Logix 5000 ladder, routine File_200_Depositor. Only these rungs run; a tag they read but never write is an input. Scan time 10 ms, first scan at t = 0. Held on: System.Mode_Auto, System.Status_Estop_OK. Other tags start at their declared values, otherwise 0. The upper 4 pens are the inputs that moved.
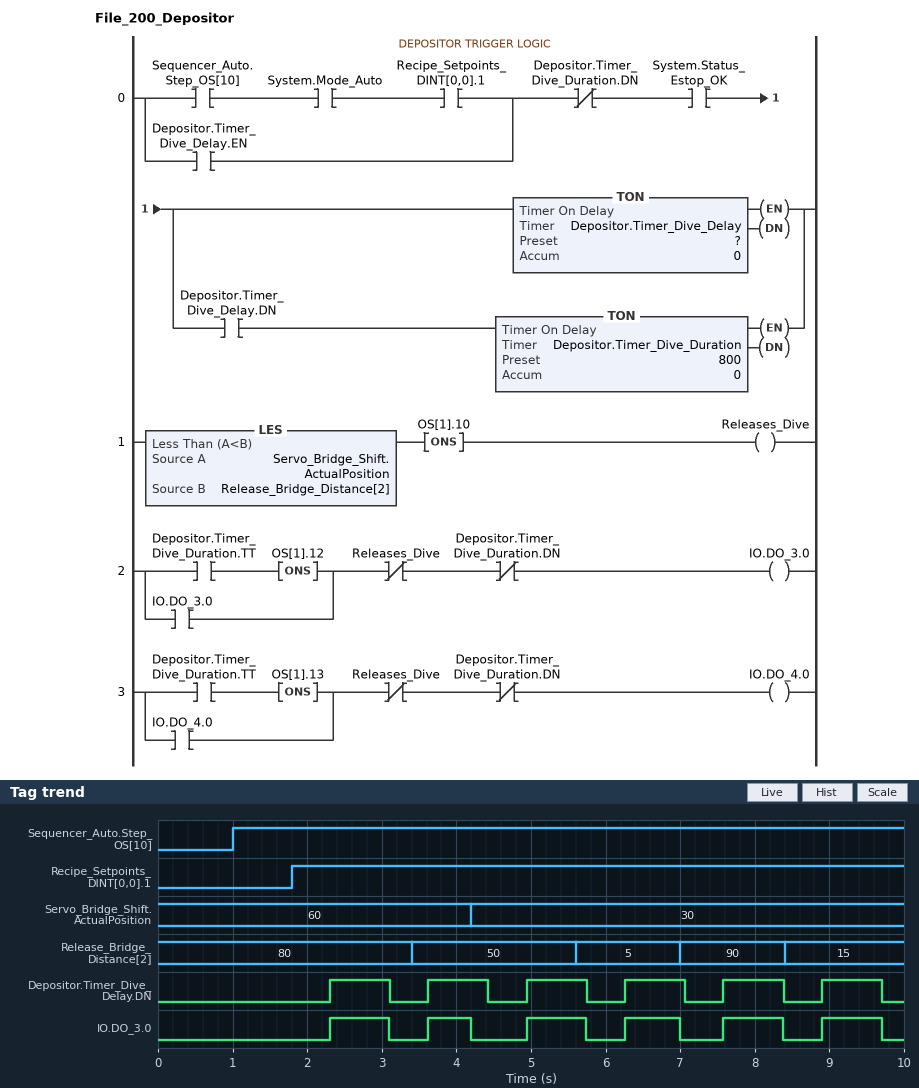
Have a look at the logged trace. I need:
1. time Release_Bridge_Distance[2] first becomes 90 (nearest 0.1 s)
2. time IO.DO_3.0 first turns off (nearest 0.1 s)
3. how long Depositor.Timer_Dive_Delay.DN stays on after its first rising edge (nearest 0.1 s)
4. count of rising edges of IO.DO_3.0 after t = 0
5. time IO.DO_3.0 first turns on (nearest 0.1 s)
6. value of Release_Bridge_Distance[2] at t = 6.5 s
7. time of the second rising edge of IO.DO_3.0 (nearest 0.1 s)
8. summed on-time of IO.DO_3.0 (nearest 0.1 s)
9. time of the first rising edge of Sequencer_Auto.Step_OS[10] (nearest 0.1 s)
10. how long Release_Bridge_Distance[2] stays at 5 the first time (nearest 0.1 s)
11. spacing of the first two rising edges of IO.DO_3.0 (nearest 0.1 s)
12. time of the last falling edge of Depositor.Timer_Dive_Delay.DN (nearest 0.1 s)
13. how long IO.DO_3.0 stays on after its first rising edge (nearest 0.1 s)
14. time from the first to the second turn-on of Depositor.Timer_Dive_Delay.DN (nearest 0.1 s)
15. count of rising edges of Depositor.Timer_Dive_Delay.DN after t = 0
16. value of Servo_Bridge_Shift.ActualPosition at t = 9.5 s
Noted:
7.0 s
3.1 s
0.8 s
6
2.3 s
5
3.6 s
4.5 s
1.0 s
1.4 s
1.3 s
9.7 s
0.8 s
1.3 s
6
30
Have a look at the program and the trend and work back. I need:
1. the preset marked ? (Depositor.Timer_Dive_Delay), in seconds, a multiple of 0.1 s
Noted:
0.5 s
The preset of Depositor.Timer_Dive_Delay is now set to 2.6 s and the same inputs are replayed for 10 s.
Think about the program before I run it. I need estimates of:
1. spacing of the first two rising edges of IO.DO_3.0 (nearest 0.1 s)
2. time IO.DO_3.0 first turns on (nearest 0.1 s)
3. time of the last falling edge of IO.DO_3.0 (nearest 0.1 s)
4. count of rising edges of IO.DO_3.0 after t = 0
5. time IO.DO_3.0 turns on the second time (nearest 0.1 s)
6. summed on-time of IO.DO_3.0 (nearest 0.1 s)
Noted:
3.4 s
4.4 s
8.6 s
2
7.8 s
1.6 s
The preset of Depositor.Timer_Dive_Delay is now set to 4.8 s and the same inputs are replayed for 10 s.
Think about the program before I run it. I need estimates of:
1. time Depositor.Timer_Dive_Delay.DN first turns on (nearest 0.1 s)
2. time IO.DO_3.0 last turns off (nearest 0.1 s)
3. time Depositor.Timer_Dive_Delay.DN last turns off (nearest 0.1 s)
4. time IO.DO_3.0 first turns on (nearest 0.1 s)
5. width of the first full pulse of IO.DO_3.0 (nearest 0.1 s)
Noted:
6.6 s
7.0 s
7.4 s
6.6 s
0.4 s
